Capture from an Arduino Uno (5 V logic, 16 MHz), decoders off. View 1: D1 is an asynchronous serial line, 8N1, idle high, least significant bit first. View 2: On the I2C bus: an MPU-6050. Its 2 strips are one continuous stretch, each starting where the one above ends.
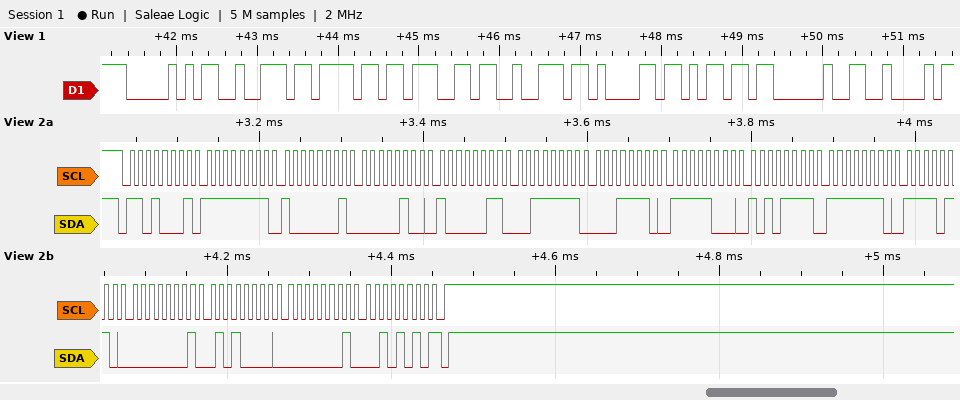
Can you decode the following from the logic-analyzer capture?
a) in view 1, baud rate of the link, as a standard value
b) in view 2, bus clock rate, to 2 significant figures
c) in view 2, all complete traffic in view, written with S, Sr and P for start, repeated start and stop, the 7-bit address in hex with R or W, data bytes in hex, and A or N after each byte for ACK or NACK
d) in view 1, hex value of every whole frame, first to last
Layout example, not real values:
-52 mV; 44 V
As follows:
9600 baud; 100 kHz; S 68R A FF A 81 A 04 A 83 A 3F A 1E A F8 A AF A FE A F6 A 01 A 50 A 01 A 2A N P; 50 72 6F 67 72 61 6D 20 42
